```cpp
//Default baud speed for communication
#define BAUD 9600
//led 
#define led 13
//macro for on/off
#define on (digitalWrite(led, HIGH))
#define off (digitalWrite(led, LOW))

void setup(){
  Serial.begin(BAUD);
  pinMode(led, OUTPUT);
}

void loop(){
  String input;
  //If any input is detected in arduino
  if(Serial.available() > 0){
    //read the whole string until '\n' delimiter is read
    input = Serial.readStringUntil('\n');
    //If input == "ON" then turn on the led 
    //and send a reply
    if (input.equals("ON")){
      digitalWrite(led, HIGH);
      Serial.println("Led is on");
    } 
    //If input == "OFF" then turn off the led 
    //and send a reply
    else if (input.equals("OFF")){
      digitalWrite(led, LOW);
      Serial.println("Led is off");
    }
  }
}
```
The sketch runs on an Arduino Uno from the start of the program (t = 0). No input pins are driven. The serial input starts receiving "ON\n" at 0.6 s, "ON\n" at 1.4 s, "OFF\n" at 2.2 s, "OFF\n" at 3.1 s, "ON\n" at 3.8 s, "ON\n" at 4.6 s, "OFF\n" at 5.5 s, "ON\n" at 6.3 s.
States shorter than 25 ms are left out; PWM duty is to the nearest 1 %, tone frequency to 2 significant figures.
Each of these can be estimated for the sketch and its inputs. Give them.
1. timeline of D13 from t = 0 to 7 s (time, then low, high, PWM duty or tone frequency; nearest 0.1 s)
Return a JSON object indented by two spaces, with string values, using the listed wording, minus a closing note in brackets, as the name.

{
  "timeline of D13 from t = 0 to 7 s": "0 s low; 0.6 s high; 2.2 s low; 3.8 s high; 5.5 s low; 6.3 s high"
}
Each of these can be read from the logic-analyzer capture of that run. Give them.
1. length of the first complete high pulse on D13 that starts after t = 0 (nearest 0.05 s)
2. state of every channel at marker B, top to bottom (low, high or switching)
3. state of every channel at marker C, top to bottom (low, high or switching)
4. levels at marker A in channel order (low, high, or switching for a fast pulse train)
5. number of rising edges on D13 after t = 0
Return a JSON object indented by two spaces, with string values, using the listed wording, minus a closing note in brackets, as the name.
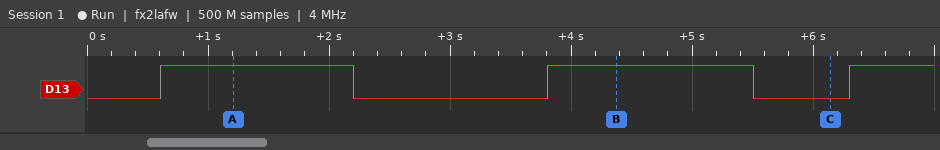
{
  "length of the first complete high pulse on D13 that starts after t = 0": "1.60 s",
  "state of every channel at marker B, top to bottom": "D13 high",
  "state of every channel at marker C, top to bottom": "D13 low",
  "levels at marker A in channel order": "D13 high",
  "number of rising edges on D13 after t = 0": "3"
}
